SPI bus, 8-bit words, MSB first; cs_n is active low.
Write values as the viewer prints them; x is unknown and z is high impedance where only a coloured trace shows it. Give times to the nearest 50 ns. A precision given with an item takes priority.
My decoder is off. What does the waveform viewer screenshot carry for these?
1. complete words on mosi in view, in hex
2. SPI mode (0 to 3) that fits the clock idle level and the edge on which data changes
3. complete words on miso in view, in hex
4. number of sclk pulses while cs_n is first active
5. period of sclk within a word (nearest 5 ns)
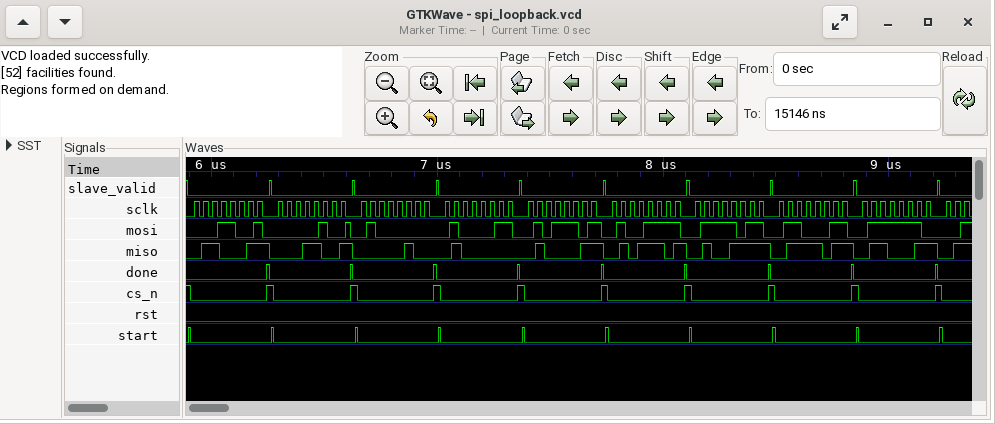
19, 04, 40, 43, 5D, 4F, 7B, 63, 7E
0
63, 19, 04, 40, 43, 5D, 4F, 7B, 63
8
40 ns
